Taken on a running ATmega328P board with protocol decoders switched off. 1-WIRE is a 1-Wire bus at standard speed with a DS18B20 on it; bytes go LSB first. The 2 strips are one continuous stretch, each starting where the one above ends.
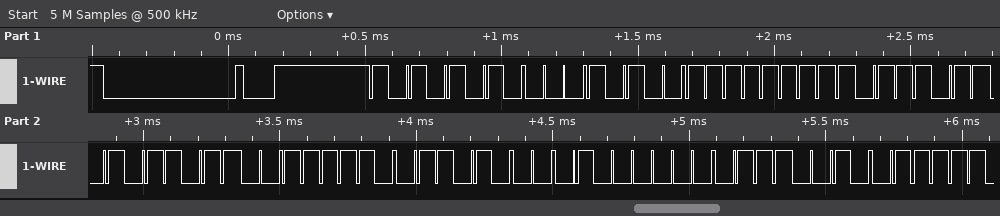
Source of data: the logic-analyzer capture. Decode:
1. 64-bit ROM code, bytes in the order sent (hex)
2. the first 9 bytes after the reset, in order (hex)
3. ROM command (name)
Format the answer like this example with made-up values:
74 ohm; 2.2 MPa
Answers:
28 FF DD DA 7C 16 02 4E; 55 28 FF DD DA 7C 16 02 4E; Match ROM
